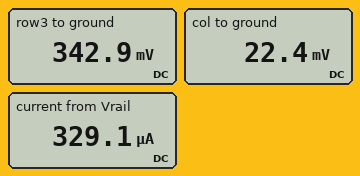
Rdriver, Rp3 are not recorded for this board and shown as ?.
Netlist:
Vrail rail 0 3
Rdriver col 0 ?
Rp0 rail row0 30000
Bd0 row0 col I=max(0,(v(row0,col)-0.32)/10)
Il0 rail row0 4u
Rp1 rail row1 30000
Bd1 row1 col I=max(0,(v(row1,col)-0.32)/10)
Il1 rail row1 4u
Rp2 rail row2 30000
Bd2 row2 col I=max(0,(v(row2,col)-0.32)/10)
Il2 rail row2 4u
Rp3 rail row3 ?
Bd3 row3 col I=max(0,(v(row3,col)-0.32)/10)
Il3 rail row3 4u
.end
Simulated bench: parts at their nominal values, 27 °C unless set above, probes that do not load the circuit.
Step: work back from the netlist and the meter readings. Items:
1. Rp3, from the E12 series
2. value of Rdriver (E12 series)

56 kΩ
68 Ω
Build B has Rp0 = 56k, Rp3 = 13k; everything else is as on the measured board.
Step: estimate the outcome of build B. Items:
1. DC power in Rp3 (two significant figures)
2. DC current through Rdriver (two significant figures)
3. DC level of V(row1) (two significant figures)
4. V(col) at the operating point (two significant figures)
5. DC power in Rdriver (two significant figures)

540 µW
440 µA
350 mV
30 mV
13 µW
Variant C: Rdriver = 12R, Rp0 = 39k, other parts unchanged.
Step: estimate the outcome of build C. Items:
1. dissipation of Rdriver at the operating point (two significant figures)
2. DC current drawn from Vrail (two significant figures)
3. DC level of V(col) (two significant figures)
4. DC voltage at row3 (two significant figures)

1.2 µW
310 µA
3.7 mV
320 mV
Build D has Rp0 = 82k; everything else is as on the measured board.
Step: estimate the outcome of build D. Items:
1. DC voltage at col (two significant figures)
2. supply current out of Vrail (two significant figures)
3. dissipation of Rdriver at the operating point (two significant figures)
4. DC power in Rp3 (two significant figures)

19 mV
270 µA
5.1 µW
130 µW
